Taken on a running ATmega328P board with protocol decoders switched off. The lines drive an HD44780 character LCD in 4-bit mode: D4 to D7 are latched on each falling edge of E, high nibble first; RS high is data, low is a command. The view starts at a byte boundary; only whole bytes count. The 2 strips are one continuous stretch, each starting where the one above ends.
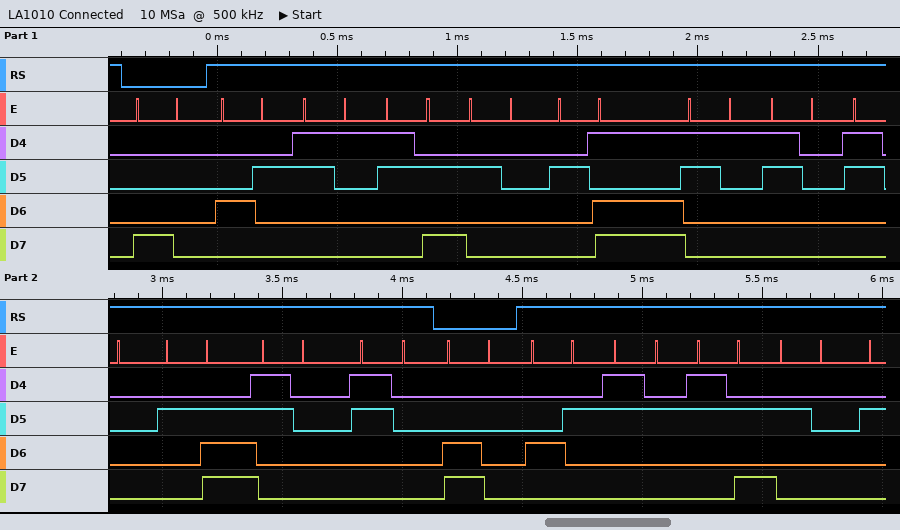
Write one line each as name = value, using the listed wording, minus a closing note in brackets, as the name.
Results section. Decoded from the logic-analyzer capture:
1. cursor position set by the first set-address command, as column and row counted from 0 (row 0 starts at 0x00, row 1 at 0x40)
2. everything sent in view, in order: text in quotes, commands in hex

cursor position set by the first set-address command, as column and row counted from 0 = column 0, row 0
everything sent in view, in order: text in quotes, commands in hex = 0x80 "B1: -100.00" 0xC0 "B2: "
